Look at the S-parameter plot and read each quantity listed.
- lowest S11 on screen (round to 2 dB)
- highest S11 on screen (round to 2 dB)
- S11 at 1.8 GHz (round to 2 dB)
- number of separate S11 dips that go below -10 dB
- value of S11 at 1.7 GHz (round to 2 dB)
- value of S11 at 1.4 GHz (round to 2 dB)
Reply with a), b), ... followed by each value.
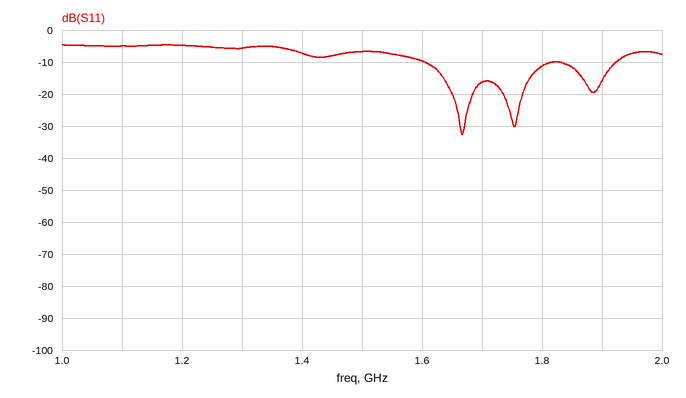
a) -32 dB
b) -4 dB
c) -12 dB
d) 3
e) -16 dB
f) -8 dB
